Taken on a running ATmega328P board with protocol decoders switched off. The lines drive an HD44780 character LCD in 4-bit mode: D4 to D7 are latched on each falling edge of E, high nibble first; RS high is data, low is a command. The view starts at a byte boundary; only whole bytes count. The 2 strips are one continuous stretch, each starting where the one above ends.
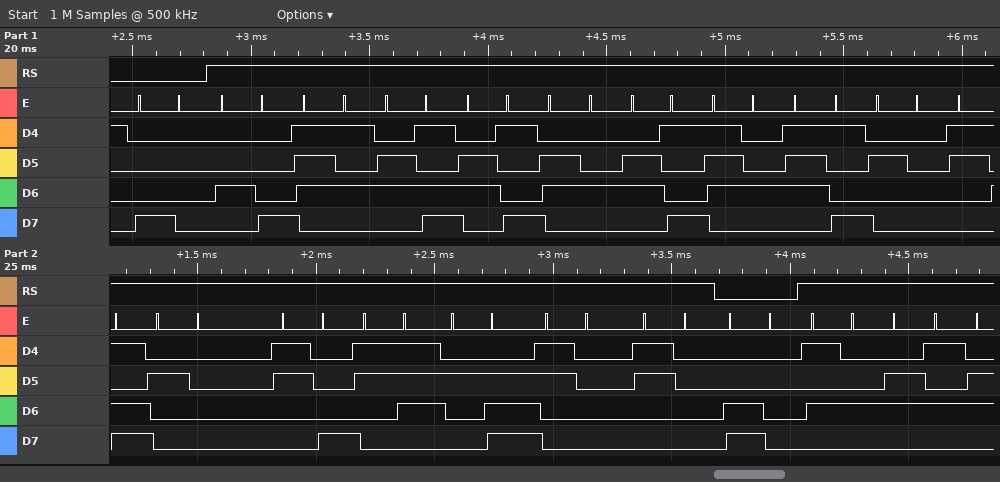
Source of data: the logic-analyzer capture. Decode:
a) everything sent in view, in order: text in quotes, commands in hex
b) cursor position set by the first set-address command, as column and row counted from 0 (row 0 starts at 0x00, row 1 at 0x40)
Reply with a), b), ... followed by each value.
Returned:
a) 0x80 "Humidity = 87.00" 0xC0 "Te"
b) column 0, row 0
